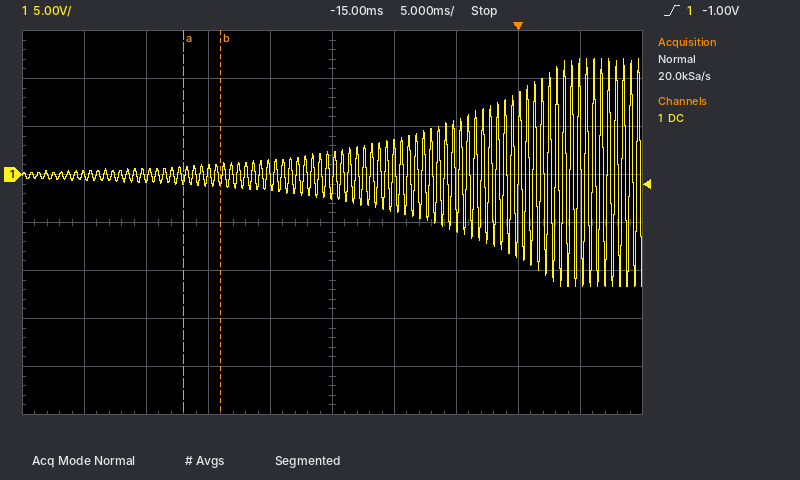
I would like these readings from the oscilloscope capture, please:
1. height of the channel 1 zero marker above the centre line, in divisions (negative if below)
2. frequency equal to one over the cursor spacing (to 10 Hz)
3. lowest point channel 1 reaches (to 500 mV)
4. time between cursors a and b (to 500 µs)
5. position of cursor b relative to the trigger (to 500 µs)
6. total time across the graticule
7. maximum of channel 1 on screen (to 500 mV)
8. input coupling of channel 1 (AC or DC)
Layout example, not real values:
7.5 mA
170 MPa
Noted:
+1.0 div
330 Hz
-11.5 V
3.0 ms
-24.0 ms
50 ms
12.0 V
DC
